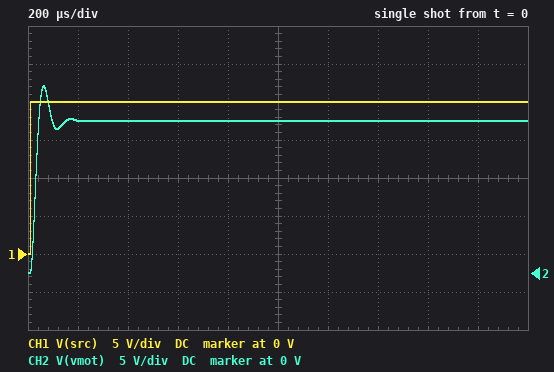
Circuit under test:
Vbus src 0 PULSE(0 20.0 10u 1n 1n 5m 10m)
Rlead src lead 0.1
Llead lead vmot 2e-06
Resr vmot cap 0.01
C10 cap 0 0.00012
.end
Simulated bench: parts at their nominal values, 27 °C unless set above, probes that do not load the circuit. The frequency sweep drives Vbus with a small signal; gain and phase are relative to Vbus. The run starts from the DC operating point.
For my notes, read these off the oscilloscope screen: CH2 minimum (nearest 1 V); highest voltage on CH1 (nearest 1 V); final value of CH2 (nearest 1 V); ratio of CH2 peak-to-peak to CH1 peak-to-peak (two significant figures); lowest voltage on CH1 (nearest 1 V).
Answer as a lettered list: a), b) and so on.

a) 0 V
b) 20 V
c) 20 V
d) 1.2
e) 0 V
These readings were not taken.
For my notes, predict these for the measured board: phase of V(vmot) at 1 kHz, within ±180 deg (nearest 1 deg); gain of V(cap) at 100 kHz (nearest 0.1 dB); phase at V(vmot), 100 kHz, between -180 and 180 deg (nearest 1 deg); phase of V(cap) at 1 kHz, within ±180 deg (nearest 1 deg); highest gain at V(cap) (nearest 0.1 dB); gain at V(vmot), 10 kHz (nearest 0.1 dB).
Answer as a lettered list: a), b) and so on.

a) -4 deg
b) -39.5 dB
c) -138 deg
d) -5 deg
e) 2.3 dB
f) 1.6 dB
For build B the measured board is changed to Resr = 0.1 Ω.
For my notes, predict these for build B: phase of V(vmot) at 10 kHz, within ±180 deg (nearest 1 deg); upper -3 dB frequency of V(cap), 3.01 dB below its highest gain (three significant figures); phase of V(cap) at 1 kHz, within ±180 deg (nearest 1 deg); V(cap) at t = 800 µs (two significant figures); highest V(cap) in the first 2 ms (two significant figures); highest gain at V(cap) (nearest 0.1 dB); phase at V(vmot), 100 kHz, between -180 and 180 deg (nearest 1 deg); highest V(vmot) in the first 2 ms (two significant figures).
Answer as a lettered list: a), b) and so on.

a) -51 deg
b) 9.30 kHz
c) -9 deg
d) 20 V
e) 20 V
f) 0 dB
g) -88 deg
h) 21 V
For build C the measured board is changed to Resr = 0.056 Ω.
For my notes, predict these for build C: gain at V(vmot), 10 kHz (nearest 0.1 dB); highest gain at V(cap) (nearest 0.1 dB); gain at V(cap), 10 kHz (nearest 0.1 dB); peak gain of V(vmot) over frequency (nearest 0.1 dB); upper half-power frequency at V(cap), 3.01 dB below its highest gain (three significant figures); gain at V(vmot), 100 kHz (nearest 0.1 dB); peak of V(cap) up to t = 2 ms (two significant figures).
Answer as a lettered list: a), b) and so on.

a) -0.7 dB
b) 0.3 dB
c) -1.4 dB
d) 0.6 dB
e) 11.4 kHz
f) -26.8 dB
g) 22 V
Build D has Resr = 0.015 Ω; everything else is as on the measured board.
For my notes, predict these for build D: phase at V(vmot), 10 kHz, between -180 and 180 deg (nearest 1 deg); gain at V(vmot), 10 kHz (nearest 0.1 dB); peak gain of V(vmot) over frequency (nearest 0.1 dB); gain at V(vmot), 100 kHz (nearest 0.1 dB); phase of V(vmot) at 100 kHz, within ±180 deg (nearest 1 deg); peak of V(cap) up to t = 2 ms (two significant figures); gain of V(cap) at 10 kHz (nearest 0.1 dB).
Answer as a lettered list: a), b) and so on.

a) -80 deg
b) 1.3 dB
c) 2.0 dB
d) -35.9 dB
e) -126 deg
f) 24 V
g) 1.2 dB
